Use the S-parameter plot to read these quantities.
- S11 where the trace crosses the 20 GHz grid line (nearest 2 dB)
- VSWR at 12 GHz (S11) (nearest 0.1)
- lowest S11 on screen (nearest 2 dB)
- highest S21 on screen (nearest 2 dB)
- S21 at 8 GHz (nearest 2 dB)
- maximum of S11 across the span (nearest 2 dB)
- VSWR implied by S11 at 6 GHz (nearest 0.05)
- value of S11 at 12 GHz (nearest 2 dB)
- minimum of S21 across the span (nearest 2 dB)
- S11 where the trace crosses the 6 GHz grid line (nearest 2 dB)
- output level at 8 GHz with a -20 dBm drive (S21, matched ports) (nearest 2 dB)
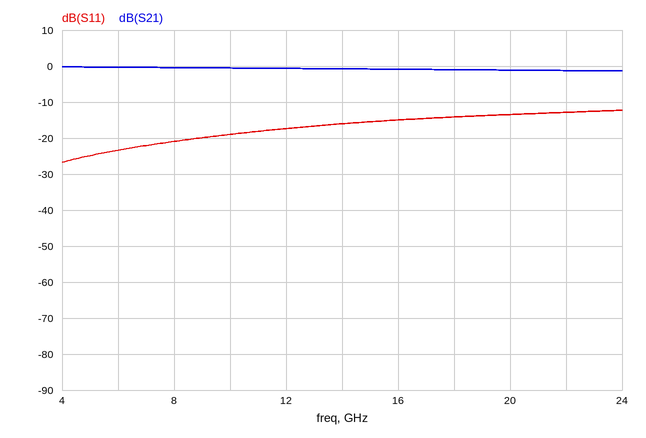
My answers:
-14 dB
1.3
-26 dB
0 dB
0 dB
-12 dB
1.15
-18 dB
-2 dB
-24 dB
-20 dBm
